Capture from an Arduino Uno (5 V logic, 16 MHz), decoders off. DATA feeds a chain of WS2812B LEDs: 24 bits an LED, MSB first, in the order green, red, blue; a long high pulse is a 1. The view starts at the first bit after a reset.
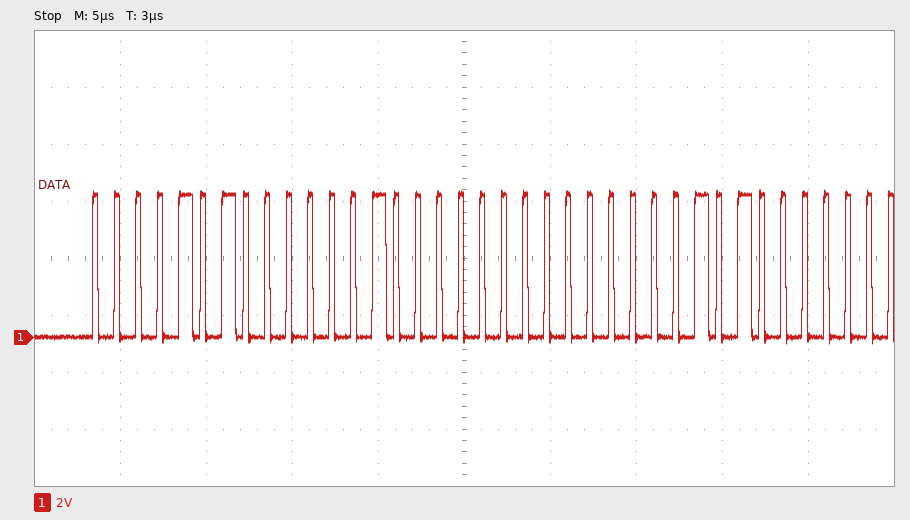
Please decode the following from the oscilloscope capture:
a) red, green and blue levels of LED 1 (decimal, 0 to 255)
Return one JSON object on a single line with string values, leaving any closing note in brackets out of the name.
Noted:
{"red, green and blue levels of LED 1": "4, 10, 0"}
